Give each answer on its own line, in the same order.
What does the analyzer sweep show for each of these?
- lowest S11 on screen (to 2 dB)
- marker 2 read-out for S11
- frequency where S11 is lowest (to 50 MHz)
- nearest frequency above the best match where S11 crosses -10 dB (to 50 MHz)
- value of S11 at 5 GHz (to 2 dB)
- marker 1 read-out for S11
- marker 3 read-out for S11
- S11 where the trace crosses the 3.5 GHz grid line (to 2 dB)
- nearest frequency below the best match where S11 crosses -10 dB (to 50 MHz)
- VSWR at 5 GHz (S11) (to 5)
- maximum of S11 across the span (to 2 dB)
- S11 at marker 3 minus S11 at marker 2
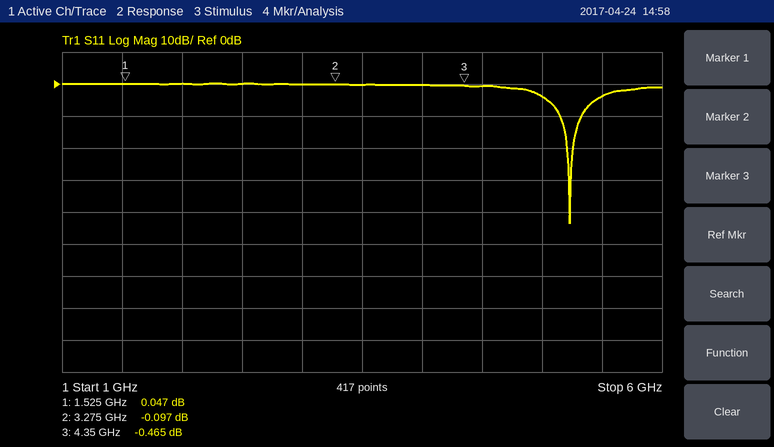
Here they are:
-44 dB
-0.097 dB
5.25 GHz
5.35 GHz
-4 dB
0.047 dB
-0.465 dB
0 dB
5.15 GHz
5
0 dB
-0.368 dB
